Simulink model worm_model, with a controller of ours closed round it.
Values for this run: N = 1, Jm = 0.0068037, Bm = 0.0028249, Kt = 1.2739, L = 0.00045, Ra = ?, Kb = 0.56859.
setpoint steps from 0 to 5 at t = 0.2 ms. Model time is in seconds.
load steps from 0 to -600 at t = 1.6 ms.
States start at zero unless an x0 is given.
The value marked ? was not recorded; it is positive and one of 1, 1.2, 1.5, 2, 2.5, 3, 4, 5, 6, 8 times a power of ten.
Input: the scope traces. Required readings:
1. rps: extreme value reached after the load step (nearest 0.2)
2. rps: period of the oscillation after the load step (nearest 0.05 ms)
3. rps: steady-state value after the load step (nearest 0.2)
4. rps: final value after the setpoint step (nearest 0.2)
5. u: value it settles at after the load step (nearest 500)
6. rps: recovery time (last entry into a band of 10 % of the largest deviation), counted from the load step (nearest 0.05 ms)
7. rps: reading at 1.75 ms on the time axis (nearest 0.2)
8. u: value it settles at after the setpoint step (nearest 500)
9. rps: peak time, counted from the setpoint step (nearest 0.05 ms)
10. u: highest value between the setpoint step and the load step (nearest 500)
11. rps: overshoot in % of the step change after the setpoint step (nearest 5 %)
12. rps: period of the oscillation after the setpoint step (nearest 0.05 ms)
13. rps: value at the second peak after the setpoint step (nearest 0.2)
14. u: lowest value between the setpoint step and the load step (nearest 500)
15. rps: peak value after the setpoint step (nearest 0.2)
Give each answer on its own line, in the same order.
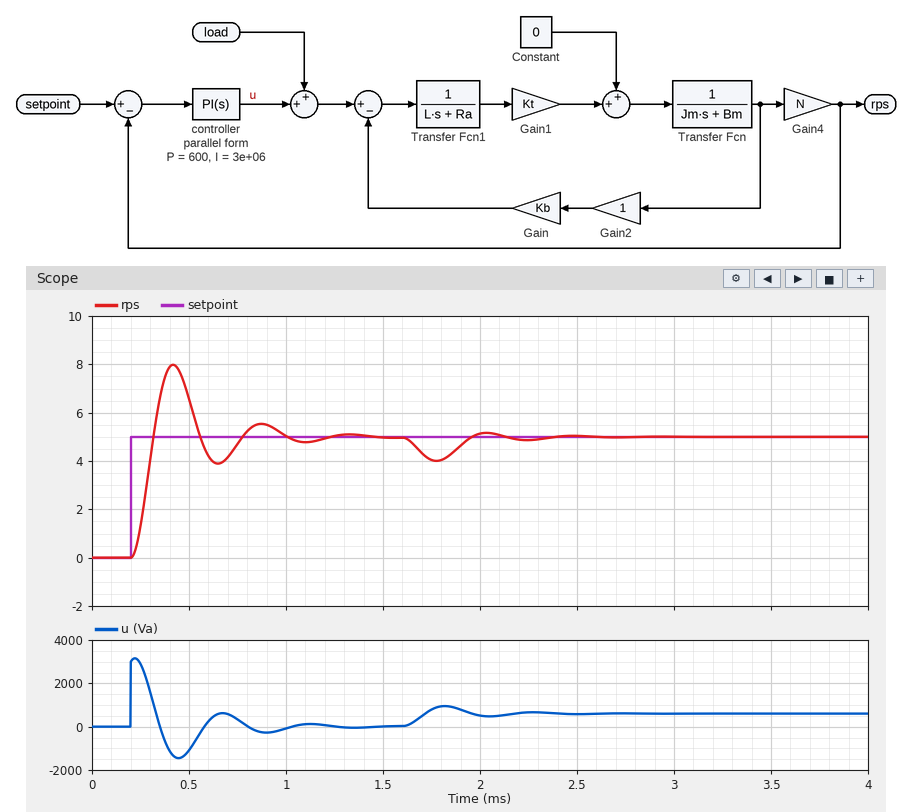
4.0
0.45 ms
5.0
5.0
500
0.70 ms
4.0
0
0.20 ms
3000
60 %
0.45 ms
5.6
-1500
8.0
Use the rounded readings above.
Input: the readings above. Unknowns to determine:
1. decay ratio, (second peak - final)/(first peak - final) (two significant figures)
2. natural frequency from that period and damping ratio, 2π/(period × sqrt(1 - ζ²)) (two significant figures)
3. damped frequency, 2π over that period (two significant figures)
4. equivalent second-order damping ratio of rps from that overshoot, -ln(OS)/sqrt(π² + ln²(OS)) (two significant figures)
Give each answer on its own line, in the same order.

0.20
14 rad/ms
14 rad/ms
0.16
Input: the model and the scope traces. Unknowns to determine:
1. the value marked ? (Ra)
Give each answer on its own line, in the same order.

6
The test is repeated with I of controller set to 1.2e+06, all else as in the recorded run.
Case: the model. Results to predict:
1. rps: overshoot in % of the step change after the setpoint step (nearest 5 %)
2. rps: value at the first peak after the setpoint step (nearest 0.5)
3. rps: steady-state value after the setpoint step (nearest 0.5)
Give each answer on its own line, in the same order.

40 %
7.0
5.0
